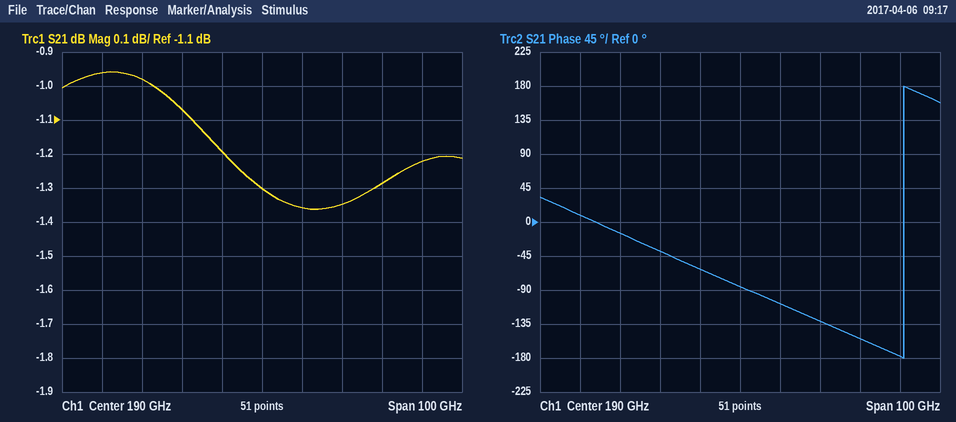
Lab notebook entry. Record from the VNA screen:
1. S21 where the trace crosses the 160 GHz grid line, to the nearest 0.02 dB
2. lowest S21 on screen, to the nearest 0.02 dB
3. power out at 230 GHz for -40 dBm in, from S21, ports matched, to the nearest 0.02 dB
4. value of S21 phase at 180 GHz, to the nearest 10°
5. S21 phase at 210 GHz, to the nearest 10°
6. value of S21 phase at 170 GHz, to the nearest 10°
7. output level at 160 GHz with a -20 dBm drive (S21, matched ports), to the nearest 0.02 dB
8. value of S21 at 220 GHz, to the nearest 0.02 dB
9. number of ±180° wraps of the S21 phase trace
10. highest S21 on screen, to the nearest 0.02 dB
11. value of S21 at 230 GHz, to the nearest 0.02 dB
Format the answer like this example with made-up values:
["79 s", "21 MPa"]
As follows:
["-0.98 dB", "-1.36 dB", "-41.22 dBm", "-60°", "-130°", "-40°", "-20.98 dBm", "-1.28 dB", "1", "-0.96 dB", "-1.22 dB"]
